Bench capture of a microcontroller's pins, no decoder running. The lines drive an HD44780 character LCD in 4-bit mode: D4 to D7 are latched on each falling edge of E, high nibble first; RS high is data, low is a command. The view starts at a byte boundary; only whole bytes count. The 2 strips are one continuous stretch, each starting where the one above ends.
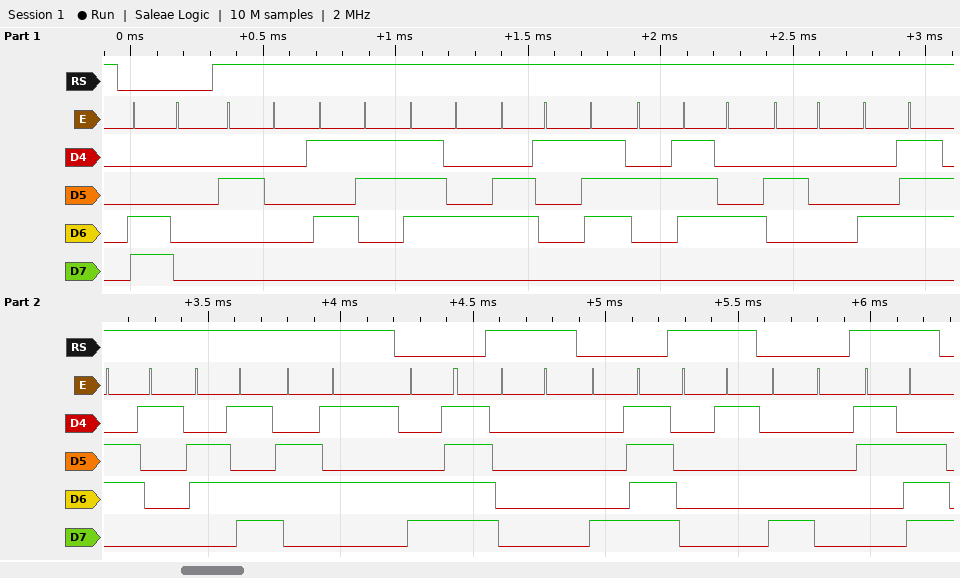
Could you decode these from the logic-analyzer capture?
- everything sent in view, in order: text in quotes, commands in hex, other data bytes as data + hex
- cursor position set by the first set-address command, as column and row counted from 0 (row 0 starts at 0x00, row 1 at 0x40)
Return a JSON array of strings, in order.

["0xC0 \" Start Game\" 0xCF data 00 0x8F data 01 0x80 \">\"", "column 0, row 1"]
